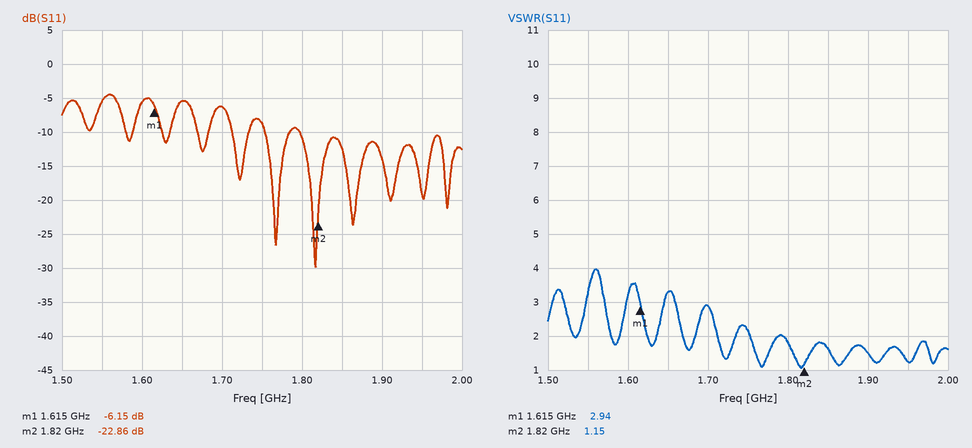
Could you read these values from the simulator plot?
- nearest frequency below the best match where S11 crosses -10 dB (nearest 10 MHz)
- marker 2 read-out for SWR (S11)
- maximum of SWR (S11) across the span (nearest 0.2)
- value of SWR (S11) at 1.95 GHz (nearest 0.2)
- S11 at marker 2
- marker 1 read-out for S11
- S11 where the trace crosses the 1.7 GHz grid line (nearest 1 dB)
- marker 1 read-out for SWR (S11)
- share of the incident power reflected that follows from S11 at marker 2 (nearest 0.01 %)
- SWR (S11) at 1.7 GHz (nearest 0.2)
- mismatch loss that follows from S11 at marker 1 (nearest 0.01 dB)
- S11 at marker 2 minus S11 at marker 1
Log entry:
1.80 GHz
1.15
4.0
1.2
-22.86 dB
-6.15 dB
-6 dB
2.94
0.52 %
2.8
1.21 dB
-16.71 dB
